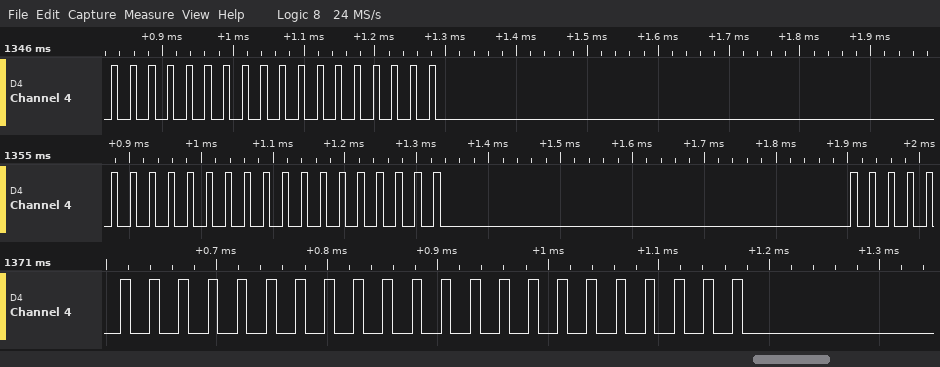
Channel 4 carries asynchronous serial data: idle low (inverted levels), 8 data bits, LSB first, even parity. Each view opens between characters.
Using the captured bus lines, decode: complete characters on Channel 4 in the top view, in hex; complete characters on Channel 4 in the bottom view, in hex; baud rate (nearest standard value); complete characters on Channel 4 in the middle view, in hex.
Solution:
DB, DB, DB, DB, FB
DB, DB, DB, DB, DB, FB
115200 baud
DB, DB, DB, DB, FB, DB
